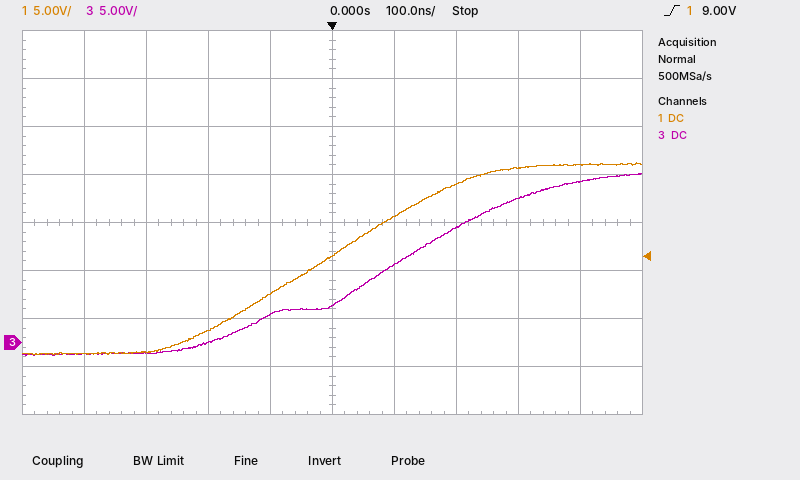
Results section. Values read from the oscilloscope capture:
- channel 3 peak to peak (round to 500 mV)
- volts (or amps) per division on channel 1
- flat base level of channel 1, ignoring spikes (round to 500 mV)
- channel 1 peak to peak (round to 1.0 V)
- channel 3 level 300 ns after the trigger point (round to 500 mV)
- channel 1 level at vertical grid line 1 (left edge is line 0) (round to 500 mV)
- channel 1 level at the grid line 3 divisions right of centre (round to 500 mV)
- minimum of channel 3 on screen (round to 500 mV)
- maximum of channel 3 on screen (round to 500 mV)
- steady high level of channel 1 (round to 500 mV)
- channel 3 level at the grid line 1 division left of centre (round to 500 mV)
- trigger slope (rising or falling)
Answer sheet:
19.0 V
5 V
-1.0 V
20.0 V
15.0 V
-1.0 V
18.0 V
-1.5 V
17.5 V
18.5 V
3.0 V
rising
